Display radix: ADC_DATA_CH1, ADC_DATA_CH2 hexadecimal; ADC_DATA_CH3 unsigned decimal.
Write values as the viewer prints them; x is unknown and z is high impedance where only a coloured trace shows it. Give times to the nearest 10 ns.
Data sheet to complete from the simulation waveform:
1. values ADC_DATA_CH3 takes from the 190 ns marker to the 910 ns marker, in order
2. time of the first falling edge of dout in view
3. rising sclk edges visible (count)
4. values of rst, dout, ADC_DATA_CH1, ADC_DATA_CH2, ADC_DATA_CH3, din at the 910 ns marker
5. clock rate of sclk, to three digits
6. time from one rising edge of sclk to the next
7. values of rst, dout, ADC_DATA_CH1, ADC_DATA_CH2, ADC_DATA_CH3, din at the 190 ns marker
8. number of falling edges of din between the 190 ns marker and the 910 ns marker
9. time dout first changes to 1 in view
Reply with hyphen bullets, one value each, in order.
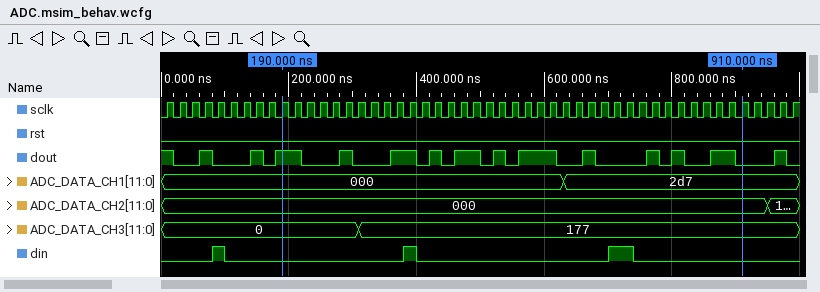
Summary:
- 0, 177
- 20 ns
- 50
- rst=0, dout=0, ADC_DATA_CH1=2d7, ADC_DATA_CH2=000, ADC_DATA_CH3=177, din=0
- 50.0 MHz
- 20 ns
- rst=0, dout=1, ADC_DATA_CH1=000, ADC_DATA_CH2=000, ADC_DATA_CH3=0, din=0
- 2
- 60 ns
